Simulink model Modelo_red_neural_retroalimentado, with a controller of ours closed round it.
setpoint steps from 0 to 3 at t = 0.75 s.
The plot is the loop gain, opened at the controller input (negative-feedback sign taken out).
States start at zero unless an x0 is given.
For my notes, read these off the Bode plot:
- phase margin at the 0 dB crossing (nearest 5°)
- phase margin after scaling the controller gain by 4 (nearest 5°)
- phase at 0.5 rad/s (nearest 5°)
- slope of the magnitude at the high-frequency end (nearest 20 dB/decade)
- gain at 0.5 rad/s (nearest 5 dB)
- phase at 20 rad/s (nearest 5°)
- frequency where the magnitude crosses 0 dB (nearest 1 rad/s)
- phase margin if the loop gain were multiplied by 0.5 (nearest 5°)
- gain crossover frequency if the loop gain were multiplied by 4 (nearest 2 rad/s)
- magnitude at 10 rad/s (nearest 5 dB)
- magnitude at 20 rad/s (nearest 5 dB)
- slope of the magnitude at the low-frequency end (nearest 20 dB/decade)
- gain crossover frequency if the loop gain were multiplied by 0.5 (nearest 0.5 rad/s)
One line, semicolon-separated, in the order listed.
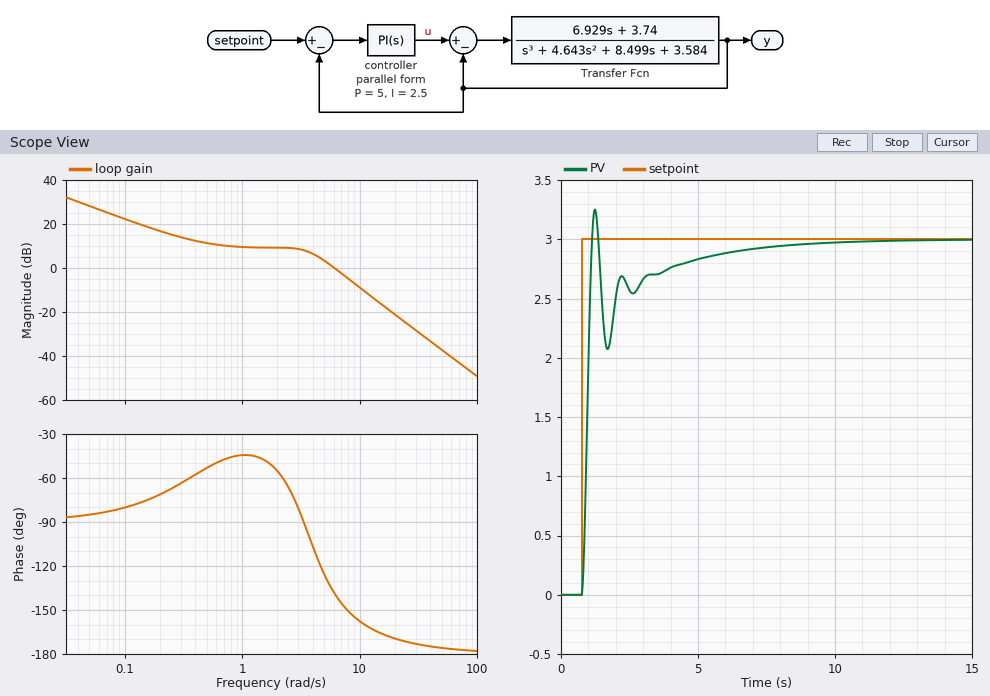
40°; 20°; -55°; -40 dB/decade; 10 dB; -170°; 6 rad/s; 70°; 12 rad/s; -10 dB; -20 dB; -20 dB/decade; 4.0 rad/s
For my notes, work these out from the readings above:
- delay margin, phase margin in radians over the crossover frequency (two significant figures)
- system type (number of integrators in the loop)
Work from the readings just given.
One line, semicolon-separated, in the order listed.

0.12 s; 1
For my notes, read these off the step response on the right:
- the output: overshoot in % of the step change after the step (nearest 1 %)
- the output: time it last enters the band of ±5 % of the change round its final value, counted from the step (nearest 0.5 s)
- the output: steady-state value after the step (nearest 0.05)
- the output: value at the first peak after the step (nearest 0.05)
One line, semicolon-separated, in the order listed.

8 %; 4.5 s; 3.00; 3.25
